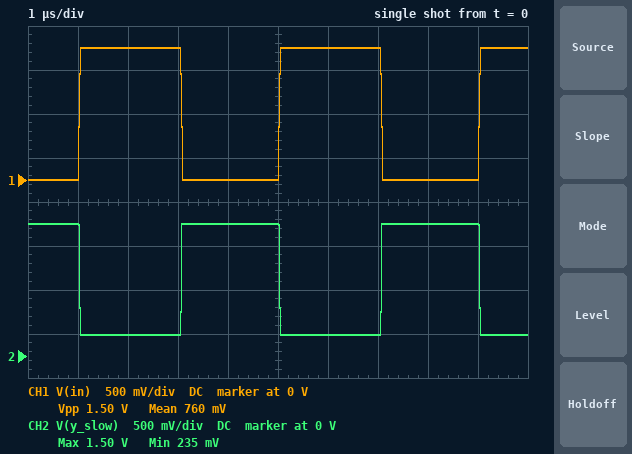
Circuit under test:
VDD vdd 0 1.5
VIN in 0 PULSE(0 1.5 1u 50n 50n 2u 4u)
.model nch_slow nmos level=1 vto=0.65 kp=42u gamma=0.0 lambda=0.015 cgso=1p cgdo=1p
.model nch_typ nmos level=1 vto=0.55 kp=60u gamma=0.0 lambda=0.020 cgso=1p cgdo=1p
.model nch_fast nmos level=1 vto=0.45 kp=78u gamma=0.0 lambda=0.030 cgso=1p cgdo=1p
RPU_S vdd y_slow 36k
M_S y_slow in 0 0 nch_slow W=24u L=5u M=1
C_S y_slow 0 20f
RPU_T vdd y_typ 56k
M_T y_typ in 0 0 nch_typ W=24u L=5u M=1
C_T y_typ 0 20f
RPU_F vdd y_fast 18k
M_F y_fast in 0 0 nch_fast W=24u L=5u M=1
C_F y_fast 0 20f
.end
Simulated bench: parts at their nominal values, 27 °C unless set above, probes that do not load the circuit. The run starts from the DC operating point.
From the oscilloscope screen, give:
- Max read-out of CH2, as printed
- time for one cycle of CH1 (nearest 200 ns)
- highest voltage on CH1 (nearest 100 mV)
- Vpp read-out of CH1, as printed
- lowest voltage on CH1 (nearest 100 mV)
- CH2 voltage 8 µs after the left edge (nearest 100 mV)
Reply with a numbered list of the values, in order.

1. 1.50 V
2. 4.0 µs
3. 1.5 V
4. 1.50 V
5. 0 V
6. 1.5 V
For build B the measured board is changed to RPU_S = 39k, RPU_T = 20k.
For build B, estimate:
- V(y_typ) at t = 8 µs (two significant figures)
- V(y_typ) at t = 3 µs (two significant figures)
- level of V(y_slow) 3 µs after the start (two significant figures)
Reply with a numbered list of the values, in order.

1. 1.5 V
2. 260 mV
3. 220 mV
